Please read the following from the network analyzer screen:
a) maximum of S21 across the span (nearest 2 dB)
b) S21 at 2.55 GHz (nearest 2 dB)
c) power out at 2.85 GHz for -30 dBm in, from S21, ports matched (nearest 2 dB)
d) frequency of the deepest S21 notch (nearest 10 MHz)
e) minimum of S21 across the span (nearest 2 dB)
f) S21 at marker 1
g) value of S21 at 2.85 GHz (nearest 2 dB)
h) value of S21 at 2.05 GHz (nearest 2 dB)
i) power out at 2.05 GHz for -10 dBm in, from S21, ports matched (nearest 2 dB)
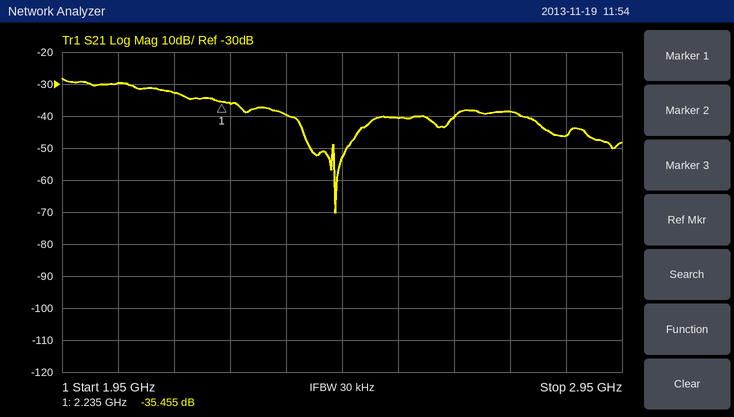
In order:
-28 dB
-40 dB
-76 dBm
2.44 GHz
-70 dB
-35.455 dB
-46 dB
-30 dB
-40 dBm
